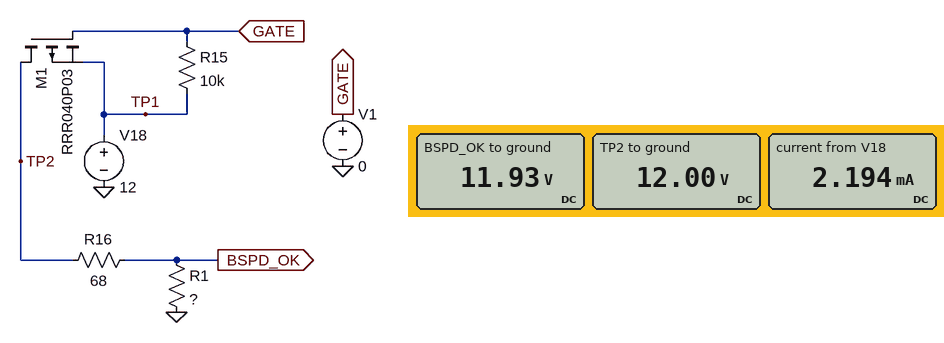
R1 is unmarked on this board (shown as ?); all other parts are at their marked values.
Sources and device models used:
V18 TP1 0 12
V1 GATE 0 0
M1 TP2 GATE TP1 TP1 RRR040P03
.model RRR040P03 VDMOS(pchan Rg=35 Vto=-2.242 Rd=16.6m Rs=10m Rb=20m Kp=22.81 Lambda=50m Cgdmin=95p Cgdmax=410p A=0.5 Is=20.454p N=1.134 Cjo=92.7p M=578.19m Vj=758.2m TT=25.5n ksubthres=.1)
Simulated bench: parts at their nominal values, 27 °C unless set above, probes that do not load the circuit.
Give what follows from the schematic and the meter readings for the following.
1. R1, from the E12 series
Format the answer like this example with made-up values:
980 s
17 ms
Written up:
12 kΩ
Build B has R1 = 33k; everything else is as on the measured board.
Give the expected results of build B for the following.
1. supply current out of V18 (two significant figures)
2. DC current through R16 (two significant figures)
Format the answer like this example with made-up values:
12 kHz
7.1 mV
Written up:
1.6 mA
360 µA
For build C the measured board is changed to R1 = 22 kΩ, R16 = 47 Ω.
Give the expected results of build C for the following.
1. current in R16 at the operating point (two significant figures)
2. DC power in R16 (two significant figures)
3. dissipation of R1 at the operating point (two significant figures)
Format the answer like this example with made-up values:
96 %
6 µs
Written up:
540 µA
14 µW
6.5 mW
